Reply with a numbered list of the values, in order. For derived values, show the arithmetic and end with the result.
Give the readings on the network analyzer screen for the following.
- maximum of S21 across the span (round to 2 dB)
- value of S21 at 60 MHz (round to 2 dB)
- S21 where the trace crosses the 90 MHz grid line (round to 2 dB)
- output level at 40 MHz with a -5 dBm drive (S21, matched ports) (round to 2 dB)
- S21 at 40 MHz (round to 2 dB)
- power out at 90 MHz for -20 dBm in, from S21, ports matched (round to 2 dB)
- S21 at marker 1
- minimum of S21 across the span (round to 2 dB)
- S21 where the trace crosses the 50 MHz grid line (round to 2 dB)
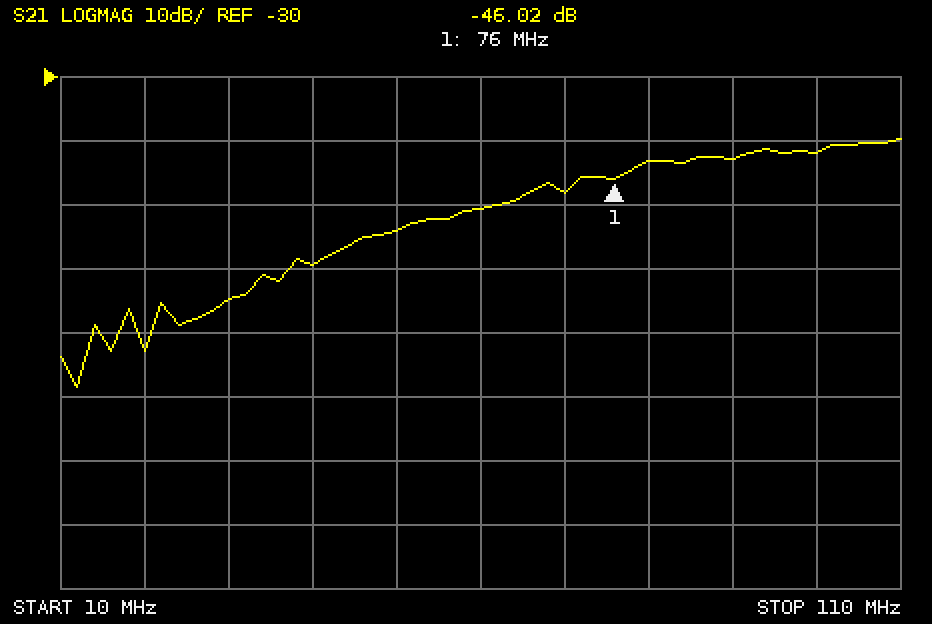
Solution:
1. -40 dB
2. -50 dB
3. -42 dB
4. -5 dBm + (-60 dB) = -64 dBm
5. -60 dB
6. -20 dBm + (-42 dB) = -62 dBm
7. -46.02 dB
8. -78 dB
9. -54 dB
